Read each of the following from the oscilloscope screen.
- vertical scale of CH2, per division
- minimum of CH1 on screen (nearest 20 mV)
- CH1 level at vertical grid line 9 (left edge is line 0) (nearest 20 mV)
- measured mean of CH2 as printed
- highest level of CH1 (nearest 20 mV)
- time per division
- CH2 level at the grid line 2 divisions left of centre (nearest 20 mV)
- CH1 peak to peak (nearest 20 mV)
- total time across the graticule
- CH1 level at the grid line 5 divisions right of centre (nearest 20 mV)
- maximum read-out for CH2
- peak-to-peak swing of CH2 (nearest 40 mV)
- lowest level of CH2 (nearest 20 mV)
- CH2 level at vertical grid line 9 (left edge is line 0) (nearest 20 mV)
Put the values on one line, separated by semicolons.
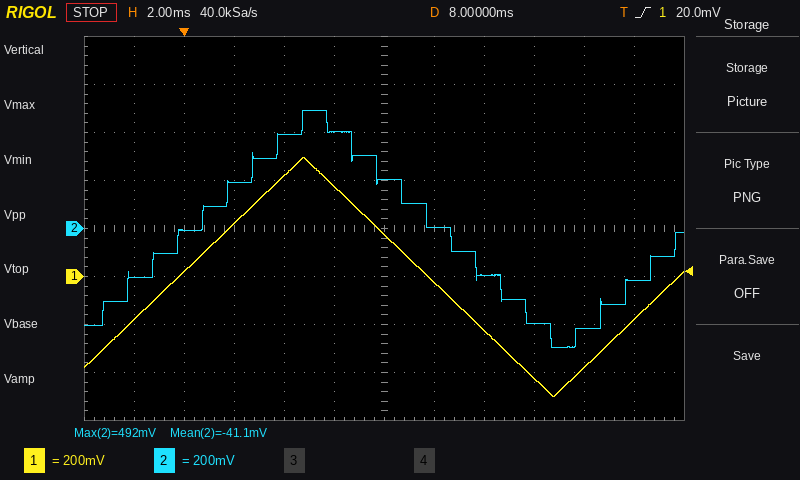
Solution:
200 mV; -500 mV; -420 mV; -41.1 mV; 500 mV; 2 ms; 400 mV; 1.00 V; 24 ms; -180 mV; 492 mV; 1.00 V; -500 mV; -400 mV
